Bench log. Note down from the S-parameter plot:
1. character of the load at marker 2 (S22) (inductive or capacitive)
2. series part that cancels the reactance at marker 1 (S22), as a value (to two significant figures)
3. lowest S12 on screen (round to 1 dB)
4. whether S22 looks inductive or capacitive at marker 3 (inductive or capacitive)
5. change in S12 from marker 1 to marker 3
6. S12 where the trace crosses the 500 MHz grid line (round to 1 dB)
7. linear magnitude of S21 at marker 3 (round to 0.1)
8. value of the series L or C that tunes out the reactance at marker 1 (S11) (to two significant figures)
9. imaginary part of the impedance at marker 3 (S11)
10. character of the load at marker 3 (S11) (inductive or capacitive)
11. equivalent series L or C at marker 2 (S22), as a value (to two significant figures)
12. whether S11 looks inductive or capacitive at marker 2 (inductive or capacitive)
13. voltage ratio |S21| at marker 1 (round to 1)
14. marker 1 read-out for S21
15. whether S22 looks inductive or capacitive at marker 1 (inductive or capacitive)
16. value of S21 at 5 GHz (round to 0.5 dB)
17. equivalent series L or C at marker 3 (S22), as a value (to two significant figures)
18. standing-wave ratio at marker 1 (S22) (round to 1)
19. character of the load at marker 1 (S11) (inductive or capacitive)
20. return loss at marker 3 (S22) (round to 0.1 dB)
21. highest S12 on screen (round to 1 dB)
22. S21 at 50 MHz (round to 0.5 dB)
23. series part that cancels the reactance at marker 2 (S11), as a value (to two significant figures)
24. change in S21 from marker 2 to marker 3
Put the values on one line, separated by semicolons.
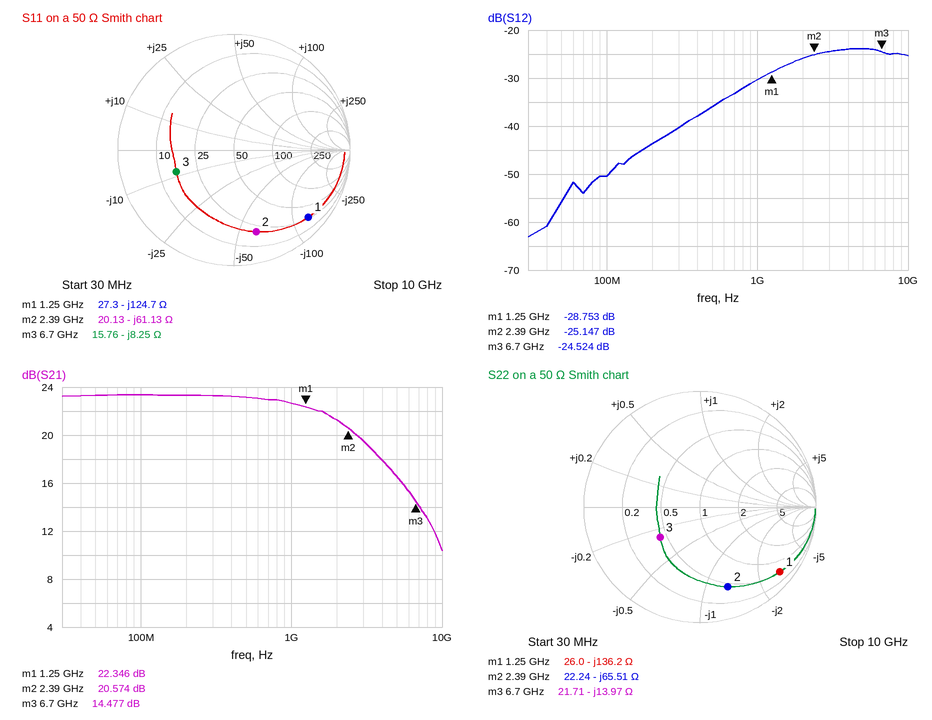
capacitive; 17 nH; -63 dB; capacitive; 4.229 dB; -36 dB; 5.3; 16 nH; -8.25 Ω; capacitive; 1.0 pF; capacitive; 13; 22.346 dB; capacitive; 16.5 dB; 1.7 pF; 17; capacitive; 7.3 dB; -24 dB; 23.5 dB; 4.1 nH; -6.097 dB
